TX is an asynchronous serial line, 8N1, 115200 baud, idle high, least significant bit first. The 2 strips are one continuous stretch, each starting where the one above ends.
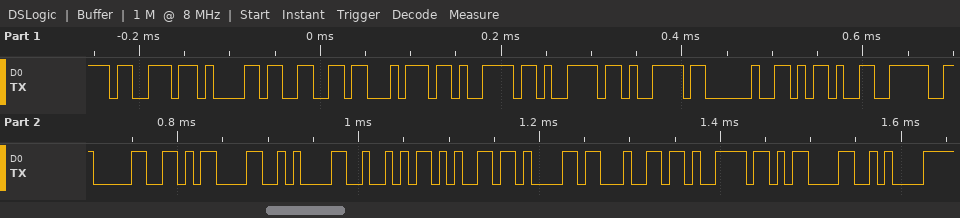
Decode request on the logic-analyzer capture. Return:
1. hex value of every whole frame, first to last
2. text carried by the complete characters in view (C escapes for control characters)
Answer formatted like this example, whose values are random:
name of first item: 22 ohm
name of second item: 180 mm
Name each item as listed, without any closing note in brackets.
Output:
hex value of every whole frame, first to last: 73 61 66 74 79 79 79 20 2D 3E 30 0D 0A 52 65 61 64 79 0D 0A
text carried by the complete characters in view: "saftyyy ->0\r\nReady\r\n"
